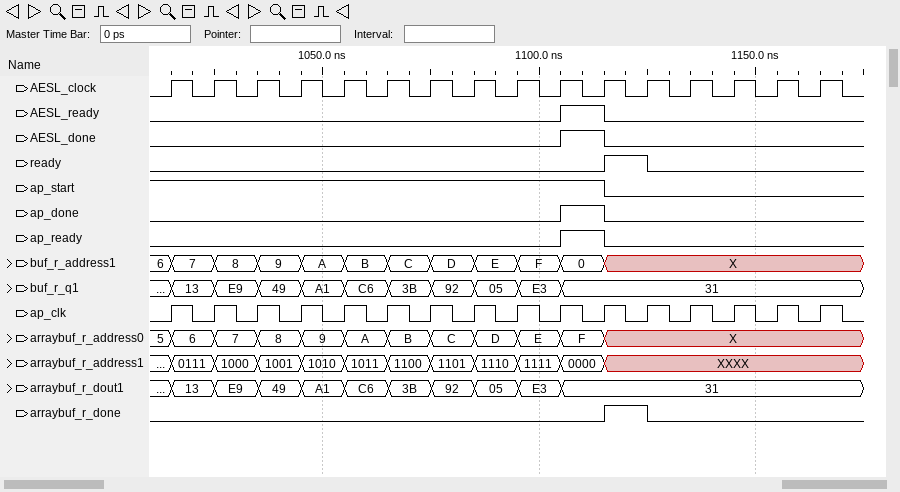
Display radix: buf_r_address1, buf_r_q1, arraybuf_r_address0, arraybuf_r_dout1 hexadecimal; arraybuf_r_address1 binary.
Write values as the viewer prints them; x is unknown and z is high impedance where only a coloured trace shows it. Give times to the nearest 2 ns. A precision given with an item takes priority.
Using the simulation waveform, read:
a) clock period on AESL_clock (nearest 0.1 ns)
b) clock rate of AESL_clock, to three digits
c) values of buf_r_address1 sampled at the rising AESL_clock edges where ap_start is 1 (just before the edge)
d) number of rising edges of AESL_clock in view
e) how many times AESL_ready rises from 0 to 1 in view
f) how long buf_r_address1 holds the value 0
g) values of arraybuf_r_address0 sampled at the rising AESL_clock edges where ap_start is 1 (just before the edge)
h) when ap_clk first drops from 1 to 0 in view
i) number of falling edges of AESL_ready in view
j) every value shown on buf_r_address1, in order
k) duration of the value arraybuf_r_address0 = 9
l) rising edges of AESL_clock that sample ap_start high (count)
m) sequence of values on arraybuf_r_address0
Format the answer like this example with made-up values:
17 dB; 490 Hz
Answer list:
10 ns; 100 MHz; 6, 7, 8, 9, A, B, C, D, E, F, 0; 16; 1; 10 ns; 5, 6, 7, 8, 9, A, B, C, D, E, F; 1020 ns; 1; 6, 7, 8, 9, A, B, C, D, E, F, 0, X; 10 ns; 11; 5, 6, 7, 8, 9, A, B, C, D, E, F, X
